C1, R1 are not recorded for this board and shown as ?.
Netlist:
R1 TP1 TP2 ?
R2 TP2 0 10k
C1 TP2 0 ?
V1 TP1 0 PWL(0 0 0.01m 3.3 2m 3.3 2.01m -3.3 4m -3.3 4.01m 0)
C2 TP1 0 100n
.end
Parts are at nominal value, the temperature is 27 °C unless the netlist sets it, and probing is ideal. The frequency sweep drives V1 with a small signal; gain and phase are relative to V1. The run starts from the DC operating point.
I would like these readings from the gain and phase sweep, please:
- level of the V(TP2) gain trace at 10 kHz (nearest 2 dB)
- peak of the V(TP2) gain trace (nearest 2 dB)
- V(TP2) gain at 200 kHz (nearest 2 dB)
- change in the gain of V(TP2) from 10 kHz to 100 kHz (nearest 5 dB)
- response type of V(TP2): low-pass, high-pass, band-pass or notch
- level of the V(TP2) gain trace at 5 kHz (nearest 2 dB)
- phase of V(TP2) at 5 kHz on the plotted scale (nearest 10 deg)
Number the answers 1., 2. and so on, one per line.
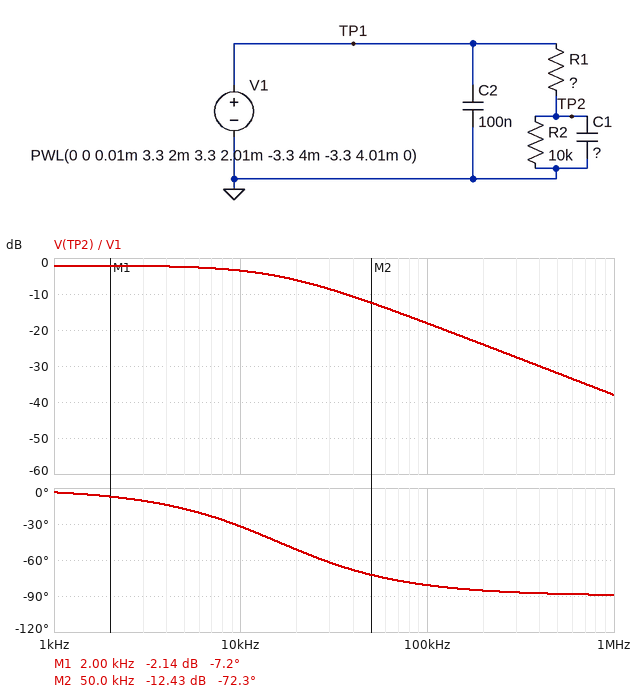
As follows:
1. -4 dB
2. -2 dB
3. -24 dB
4. -15 dB
5. low-pass
6. -2 dB
7. -20 deg
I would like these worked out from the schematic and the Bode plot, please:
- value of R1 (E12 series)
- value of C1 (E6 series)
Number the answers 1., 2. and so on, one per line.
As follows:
1. 2.7 kΩ
2. 4.7 nF
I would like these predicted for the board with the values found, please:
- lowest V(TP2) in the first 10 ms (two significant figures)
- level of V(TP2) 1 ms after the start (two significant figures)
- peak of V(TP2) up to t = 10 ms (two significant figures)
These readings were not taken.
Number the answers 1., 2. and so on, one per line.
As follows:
1. -2.6 V
2. 2.6 V
3. 2.6 V
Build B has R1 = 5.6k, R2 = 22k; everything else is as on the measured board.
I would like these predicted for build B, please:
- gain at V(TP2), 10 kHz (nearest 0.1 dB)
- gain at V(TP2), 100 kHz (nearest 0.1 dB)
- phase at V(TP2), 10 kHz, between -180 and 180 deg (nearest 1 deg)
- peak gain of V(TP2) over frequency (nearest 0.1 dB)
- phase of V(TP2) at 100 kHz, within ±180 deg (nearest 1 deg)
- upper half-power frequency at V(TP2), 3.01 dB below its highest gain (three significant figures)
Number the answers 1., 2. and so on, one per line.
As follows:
1. -6.3 dB
2. -24.4 dB
3. -53 deg
4. -2.0 dB
5. -86 deg
6. 7.59 kHz
